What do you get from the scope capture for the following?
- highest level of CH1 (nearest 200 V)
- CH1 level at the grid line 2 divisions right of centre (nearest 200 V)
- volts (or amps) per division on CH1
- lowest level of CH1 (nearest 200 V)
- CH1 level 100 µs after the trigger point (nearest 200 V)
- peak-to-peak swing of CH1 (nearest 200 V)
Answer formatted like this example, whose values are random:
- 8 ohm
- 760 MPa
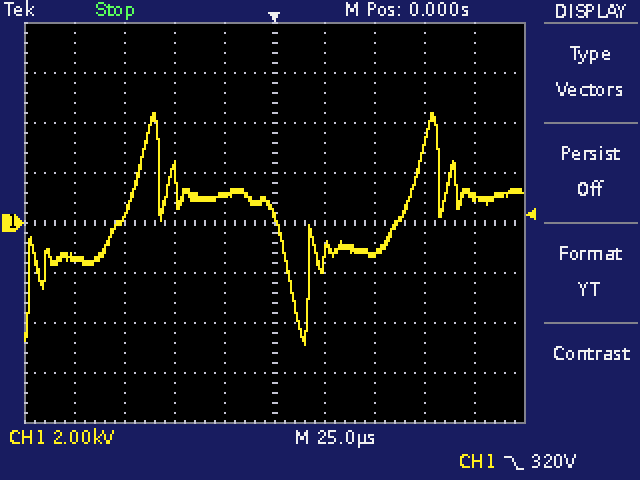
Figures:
- 4.4 kV
- -1.2 kV
- 2 kV
- -4.8 kV
- 1.0 kV
- 9.2 kV
